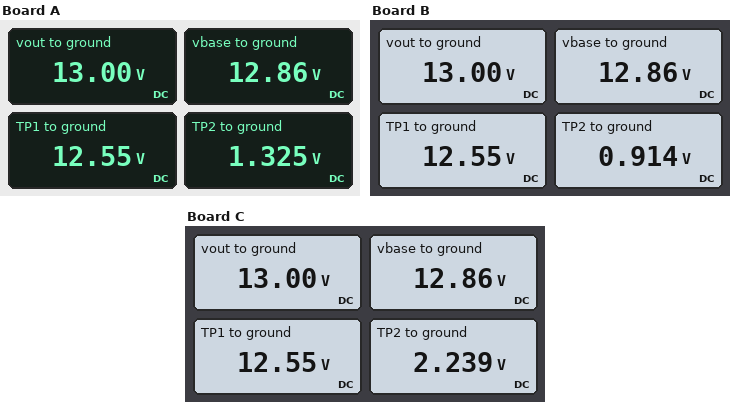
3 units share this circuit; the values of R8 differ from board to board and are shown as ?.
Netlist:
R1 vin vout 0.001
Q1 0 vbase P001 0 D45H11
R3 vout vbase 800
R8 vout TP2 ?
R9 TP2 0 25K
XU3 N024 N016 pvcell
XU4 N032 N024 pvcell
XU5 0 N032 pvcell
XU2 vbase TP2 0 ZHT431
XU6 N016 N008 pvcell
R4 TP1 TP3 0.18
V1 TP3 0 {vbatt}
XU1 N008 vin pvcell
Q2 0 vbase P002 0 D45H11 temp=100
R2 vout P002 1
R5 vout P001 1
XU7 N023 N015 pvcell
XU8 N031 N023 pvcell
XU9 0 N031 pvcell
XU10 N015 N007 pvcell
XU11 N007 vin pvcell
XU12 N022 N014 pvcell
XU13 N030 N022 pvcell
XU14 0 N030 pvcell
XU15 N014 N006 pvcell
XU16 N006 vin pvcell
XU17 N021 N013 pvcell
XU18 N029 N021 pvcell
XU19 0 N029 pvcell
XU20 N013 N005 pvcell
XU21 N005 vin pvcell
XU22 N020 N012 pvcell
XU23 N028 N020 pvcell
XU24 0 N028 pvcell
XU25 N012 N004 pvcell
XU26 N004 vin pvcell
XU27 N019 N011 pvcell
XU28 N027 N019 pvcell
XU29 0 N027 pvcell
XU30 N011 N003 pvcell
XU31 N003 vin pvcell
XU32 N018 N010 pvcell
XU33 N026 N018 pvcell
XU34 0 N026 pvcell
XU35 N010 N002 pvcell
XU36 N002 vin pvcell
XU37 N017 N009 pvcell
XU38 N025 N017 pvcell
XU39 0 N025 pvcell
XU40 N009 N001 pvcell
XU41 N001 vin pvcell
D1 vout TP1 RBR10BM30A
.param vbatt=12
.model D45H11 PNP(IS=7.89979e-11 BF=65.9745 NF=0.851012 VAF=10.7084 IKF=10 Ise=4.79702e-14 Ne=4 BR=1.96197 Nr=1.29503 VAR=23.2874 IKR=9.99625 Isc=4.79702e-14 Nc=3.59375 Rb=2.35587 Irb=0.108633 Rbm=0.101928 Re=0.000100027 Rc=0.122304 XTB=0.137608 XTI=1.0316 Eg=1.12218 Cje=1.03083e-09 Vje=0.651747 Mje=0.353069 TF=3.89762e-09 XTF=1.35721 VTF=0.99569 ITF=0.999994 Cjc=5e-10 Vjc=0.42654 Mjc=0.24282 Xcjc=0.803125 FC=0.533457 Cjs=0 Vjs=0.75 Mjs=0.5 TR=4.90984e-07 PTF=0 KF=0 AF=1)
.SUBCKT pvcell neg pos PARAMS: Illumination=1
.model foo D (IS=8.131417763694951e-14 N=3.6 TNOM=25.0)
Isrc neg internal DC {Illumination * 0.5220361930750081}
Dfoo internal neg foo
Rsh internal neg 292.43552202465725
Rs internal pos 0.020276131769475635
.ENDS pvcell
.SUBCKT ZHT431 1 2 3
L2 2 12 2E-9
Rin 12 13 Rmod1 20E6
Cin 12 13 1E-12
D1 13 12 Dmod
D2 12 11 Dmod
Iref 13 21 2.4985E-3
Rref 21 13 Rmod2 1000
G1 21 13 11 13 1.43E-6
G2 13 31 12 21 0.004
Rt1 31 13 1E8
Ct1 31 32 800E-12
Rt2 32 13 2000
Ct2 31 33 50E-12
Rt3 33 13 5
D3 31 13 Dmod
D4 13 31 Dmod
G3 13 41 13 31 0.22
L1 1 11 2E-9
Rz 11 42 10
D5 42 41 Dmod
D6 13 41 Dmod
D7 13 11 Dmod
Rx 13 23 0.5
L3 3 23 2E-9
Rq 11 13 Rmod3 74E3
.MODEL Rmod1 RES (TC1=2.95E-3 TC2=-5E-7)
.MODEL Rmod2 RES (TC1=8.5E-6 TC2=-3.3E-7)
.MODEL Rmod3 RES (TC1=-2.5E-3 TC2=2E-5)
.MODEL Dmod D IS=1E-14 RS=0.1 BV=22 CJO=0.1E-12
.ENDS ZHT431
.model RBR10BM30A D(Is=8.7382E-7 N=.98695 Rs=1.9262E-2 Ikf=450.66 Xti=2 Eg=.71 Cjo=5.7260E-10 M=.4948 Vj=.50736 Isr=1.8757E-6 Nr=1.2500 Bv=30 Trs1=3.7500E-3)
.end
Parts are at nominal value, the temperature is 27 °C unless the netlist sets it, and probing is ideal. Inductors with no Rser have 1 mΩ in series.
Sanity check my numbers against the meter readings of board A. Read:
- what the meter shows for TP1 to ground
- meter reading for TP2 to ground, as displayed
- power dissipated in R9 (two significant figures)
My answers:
12.55 V
1.325 V
70 µW
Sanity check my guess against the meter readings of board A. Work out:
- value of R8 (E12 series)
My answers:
220 kΩ
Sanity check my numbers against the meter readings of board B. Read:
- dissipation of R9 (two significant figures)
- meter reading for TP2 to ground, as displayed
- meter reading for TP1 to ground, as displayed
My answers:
33 µW
0.914 V
12.55 V
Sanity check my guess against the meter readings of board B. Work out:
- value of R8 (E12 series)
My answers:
330 kΩ
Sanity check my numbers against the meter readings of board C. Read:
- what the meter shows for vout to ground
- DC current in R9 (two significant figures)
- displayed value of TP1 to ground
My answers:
13.00 V
90 µA
12.55 V
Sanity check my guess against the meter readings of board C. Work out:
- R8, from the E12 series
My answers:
120 kΩ
